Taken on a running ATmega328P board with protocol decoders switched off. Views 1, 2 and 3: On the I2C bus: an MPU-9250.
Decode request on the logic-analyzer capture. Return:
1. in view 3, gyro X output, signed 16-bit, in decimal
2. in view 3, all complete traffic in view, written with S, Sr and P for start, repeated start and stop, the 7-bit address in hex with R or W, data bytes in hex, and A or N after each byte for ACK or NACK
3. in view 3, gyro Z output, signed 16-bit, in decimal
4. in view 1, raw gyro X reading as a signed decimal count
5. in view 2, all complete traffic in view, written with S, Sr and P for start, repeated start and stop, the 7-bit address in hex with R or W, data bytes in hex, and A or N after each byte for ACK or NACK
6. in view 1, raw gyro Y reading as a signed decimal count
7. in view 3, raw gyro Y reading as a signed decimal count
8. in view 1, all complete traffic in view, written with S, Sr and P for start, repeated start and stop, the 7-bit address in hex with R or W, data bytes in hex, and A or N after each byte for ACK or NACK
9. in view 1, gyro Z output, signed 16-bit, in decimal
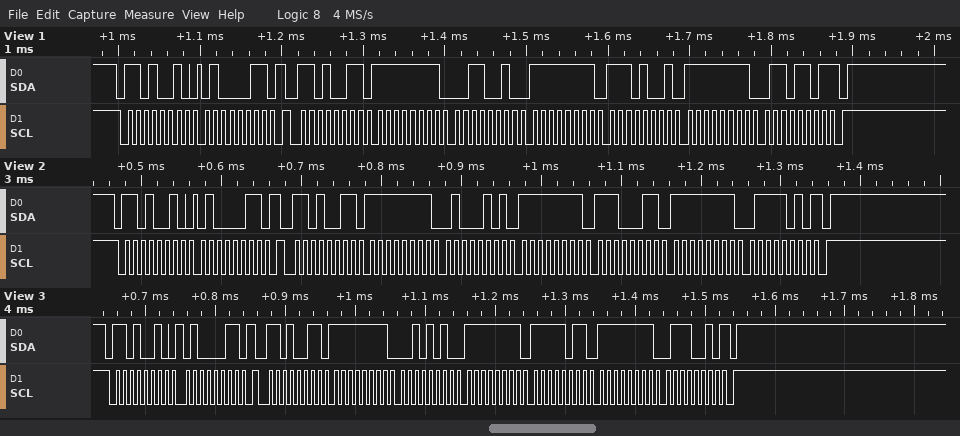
-214
S 69W A 43 A Sr 69R A FF A 2A A FF A FB A FF A 72 N P
-142
-206
S 69W A 43 A Sr 69R A FF A 45 A FF A E3 A FF A 7A N P
-23
-5
S 69W A 43 A Sr 69R A FF A 32 A FF A E9 A FF A 6D N P
-147
